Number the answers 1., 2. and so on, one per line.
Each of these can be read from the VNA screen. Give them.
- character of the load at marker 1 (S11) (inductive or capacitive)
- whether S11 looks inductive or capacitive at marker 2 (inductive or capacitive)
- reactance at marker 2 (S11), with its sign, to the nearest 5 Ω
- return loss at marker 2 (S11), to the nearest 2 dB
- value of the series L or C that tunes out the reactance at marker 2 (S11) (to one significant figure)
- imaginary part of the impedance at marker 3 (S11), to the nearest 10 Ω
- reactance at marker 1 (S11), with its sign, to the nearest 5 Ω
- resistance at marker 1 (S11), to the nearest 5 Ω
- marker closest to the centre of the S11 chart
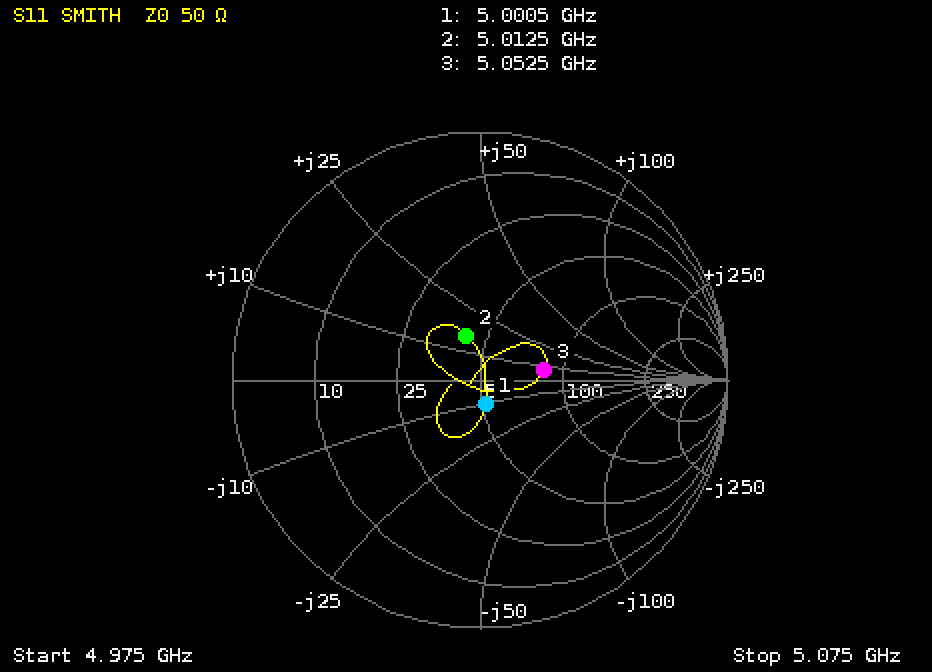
1. capacitive
2. inductive
3. +15 Ω
4. 14 dB
5. 2 pF
6. +10 Ω
7. -10 Ω
8. 50 Ω
9. marker 1
